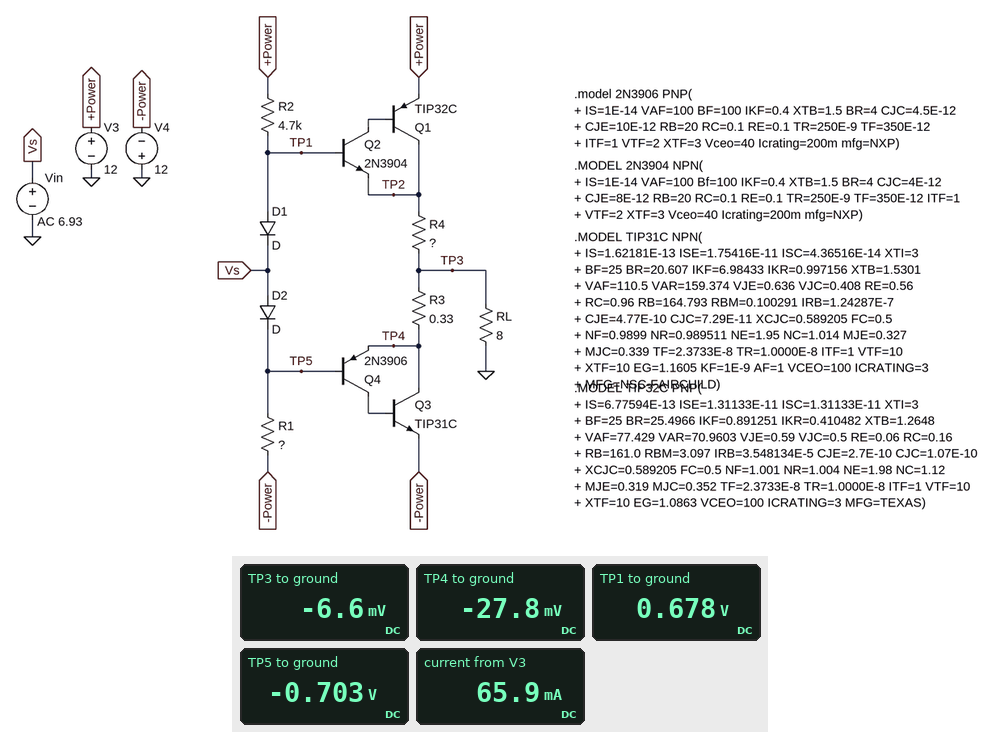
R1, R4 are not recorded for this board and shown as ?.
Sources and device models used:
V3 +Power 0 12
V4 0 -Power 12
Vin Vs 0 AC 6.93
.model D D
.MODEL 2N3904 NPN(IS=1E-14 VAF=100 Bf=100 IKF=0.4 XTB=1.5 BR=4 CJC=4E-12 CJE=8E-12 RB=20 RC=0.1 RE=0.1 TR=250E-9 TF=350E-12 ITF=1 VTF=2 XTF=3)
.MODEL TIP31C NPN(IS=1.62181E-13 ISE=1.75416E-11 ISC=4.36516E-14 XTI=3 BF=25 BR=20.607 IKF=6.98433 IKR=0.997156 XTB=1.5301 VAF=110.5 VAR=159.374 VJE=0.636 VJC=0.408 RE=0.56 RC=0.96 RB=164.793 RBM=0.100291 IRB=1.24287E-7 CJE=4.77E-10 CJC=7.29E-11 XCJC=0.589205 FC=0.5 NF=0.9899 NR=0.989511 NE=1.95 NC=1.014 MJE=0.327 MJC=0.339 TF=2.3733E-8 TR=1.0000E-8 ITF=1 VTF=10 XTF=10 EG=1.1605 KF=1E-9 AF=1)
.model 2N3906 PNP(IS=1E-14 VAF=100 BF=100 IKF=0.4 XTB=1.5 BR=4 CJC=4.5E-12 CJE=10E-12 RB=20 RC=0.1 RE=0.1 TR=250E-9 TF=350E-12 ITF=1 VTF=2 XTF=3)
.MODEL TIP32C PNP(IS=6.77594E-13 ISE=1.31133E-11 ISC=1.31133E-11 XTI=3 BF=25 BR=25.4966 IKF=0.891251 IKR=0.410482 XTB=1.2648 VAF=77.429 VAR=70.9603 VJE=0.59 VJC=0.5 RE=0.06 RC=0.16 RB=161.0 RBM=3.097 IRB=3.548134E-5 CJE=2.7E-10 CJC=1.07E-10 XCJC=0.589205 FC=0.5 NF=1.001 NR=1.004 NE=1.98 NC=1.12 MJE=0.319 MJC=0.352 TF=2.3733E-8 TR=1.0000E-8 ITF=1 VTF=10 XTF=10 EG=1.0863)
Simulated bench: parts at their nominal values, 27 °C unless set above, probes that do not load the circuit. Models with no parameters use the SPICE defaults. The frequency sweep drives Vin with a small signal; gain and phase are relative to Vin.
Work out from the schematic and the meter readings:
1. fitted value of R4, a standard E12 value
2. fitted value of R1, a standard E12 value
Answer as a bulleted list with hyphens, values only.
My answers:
- 0.15 Ω
- 1.8 kΩ
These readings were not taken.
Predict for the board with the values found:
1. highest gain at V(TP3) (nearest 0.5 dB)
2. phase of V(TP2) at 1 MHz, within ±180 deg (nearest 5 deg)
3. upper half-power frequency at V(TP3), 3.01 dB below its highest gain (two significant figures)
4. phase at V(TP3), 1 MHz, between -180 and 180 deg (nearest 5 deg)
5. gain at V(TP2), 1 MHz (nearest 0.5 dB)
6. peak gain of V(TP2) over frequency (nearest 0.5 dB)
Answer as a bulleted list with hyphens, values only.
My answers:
- -0.5 dB
- -5 deg
- 7.4 MHz
- -5 deg
- -0.5 dB
- -0.5 dB
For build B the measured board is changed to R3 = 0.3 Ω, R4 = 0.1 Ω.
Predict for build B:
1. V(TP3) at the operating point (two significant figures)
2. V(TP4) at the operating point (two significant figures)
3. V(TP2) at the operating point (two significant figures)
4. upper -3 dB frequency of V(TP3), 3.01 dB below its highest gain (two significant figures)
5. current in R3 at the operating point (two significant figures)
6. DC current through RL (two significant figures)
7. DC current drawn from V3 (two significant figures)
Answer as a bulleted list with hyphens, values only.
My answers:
- -5.6 mV
- -26 mV
- 1.1 mV
- 8.0 MHz
- 68 mA
- 700 µA
- 70 mA
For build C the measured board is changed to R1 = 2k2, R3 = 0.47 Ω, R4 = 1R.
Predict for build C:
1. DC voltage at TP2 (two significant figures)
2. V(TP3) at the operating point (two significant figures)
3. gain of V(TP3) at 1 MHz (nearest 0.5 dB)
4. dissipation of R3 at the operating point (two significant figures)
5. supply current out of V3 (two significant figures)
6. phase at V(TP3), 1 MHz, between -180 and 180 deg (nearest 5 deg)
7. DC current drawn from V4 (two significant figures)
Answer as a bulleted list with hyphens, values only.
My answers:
- 18 mV
- -18 mV
- -1.0 dB
- 700 µW
- 39 mA
- -10 deg
- 44 mA
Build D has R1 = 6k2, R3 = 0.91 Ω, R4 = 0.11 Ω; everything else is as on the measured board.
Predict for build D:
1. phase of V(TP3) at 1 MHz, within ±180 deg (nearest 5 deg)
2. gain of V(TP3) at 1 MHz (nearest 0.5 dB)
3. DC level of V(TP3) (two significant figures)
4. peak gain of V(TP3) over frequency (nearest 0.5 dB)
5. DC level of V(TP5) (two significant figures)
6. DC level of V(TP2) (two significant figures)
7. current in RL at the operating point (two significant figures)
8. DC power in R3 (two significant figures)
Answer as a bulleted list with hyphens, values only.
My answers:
- -10 deg
- -1.0 dB
- 16 mV
- -0.5 dB
- -670 mV
- 20 mV
- 2.0 mA
- 970 µW
